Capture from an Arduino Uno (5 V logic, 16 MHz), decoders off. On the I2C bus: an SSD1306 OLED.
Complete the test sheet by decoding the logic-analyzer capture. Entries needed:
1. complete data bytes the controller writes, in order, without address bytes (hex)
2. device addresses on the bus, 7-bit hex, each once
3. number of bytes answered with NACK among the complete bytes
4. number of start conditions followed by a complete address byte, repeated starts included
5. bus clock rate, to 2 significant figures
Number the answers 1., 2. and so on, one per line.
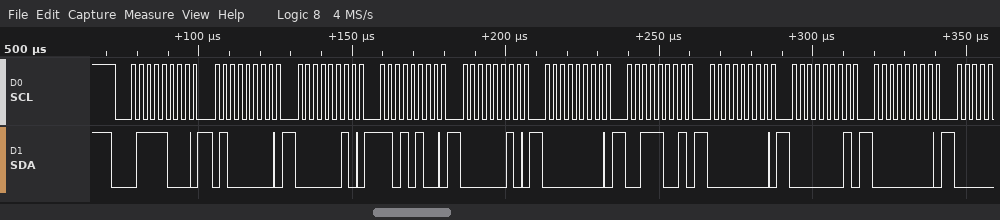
1. 40 02 D4 02 00 39 00 01 00
2. 0x3C
3. 0
4. 1
5. 400 kHz
